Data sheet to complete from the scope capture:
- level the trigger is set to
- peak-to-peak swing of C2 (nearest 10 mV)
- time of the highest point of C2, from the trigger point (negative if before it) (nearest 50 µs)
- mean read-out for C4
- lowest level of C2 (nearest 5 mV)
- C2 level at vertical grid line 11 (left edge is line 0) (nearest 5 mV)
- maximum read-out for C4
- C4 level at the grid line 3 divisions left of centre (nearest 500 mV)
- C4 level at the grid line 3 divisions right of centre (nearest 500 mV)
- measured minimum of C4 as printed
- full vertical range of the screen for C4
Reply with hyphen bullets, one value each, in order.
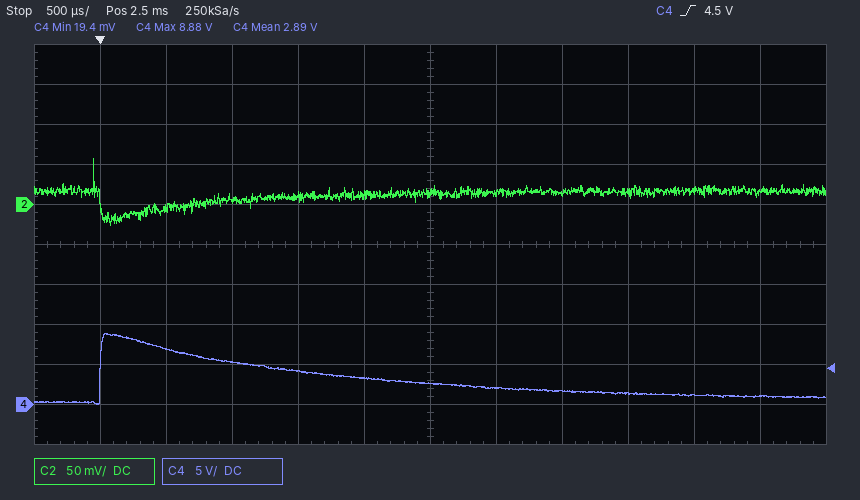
- 4.5 V
- 80 mV
- -50 µs
- 2.89 V
- -25 mV
- 15 mV
- 8.88 V
- 5.5 V
- 1.5 V
- 19.4 mV
- 50 V
